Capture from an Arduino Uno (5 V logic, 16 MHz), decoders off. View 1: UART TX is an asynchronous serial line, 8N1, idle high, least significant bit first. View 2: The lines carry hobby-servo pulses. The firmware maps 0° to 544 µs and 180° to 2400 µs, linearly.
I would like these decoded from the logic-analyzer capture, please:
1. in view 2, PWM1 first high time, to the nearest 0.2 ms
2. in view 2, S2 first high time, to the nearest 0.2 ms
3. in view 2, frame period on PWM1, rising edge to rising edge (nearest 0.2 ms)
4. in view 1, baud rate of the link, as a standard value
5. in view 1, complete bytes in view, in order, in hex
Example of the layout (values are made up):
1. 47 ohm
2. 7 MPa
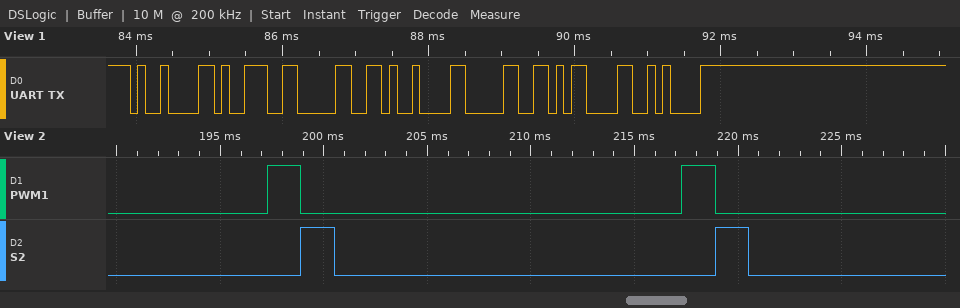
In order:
1. 1.6 ms
2. 1.6 ms
3. 20.0 ms
4. 9600 baud
5. 09 39 30 09 30 0D 0A
